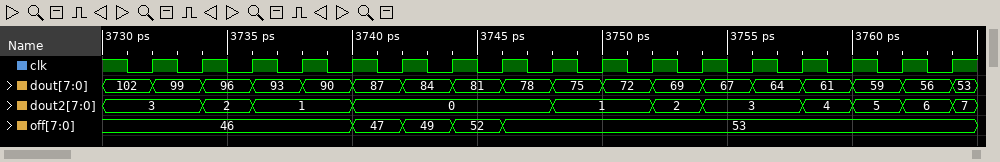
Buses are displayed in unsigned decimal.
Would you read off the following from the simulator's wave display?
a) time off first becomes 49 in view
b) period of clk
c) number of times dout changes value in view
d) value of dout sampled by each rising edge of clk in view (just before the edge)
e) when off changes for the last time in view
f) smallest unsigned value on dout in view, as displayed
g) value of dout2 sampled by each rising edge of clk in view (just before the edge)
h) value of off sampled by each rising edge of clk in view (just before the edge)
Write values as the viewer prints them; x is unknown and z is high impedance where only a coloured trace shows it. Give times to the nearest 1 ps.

3742 ps
2 ps
17
102, 99, 96, 93, 90, 87, 84, 81, 78, 75, 72, 69, 67, 64, 61, 59, 56
3746 ps
53
3, 3, 2, 1, 1, 0, 0, 0, 0, 1, 1, 2, 3, 3, 4, 5, 6
46, 46, 46, 46, 46, 47, 49, 52, 53, 53, 53, 53, 53, 53, 53, 53, 53
